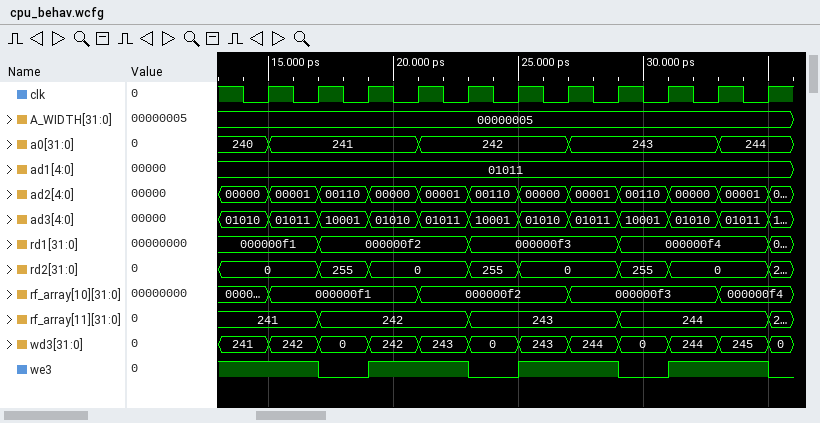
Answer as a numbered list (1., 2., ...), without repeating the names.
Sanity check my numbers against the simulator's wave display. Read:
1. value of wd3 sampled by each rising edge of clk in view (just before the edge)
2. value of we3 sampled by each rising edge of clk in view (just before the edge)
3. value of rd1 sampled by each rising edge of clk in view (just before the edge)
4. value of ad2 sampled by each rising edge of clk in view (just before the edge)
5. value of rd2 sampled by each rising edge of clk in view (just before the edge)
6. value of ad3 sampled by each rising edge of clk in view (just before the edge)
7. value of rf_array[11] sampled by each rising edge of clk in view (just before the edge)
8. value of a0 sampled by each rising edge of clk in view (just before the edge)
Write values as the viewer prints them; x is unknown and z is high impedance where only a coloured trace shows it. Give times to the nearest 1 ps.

1. 241, 242, 0, 242, 243, 0, 243, 244, 0, 244, 245
2. 1 1 0 1 1 0 1 1 0 1 1
3. 000000f1, 000000f1, 000000f2, 000000f2, 000000f2, 000000f3, 000000f3, 000000f3, 000000f4, 000000f4, 000000f4
4. 00000, 00001, 00110, 00000, 00001, 00110, 00000, 00001, 00110, 00000, 00001
5. 0, 0, 255, 0, 0, 255, 0, 0, 255, 0, 0
6. 01010, 01011, 10001, 01010, 01011, 10001, 01010, 01011, 10001, 01010, 01011
7. 241, 241, 242, 242, 242, 243, 243, 243, 244, 244, 244
8. 240, 241, 241, 241, 242, 242, 242, 243, 243, 243, 244
